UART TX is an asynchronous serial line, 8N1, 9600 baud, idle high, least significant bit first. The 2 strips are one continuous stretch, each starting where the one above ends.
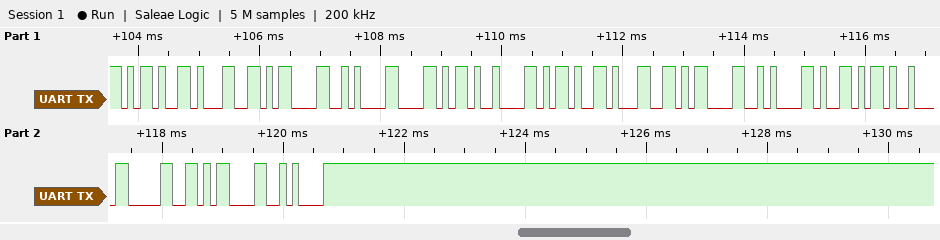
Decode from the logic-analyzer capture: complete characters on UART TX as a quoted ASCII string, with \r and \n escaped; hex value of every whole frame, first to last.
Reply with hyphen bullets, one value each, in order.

- "-1\r\nX\t-1\r\nY\t0\r\n"
- 2D 31 0D 0A 58 09 2D 31 0D 0A 59 09 30 0D 0A
